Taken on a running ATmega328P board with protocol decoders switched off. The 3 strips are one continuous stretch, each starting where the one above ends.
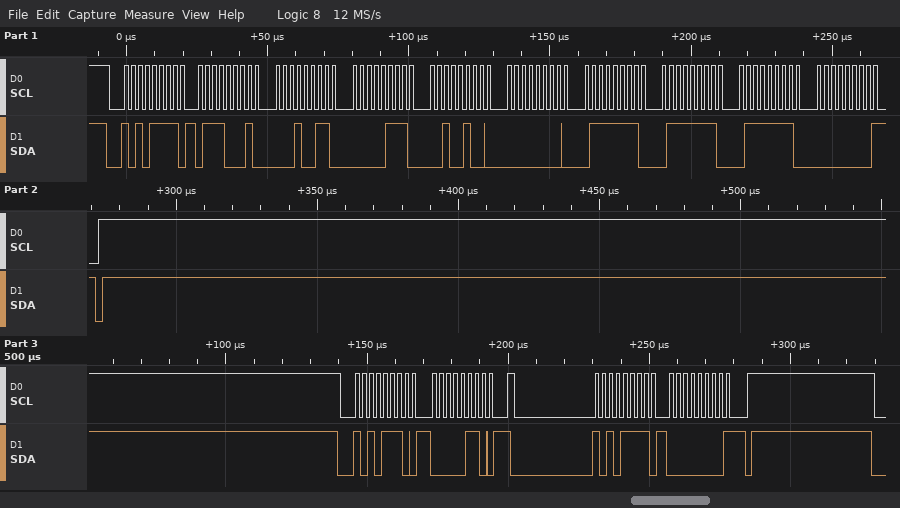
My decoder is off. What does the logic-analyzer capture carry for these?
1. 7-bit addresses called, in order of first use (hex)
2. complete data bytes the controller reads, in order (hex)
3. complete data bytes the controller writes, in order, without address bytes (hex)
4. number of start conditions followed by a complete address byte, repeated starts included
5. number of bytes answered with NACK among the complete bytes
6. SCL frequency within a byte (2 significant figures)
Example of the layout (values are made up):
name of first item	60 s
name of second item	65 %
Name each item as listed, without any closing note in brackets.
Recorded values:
7-bit addresses called, in order of first use	0x57
complete data bytes the controller reads, in order	71 13 07 24 00 7F 7F 7F 00 00
complete data bytes the controller writes, in order, without address bytes	06
number of start conditions followed by a complete address byte, repeated starts included	3
number of bytes answered with NACK among the complete bytes	2
SCL frequency within a byte	400 kHz
